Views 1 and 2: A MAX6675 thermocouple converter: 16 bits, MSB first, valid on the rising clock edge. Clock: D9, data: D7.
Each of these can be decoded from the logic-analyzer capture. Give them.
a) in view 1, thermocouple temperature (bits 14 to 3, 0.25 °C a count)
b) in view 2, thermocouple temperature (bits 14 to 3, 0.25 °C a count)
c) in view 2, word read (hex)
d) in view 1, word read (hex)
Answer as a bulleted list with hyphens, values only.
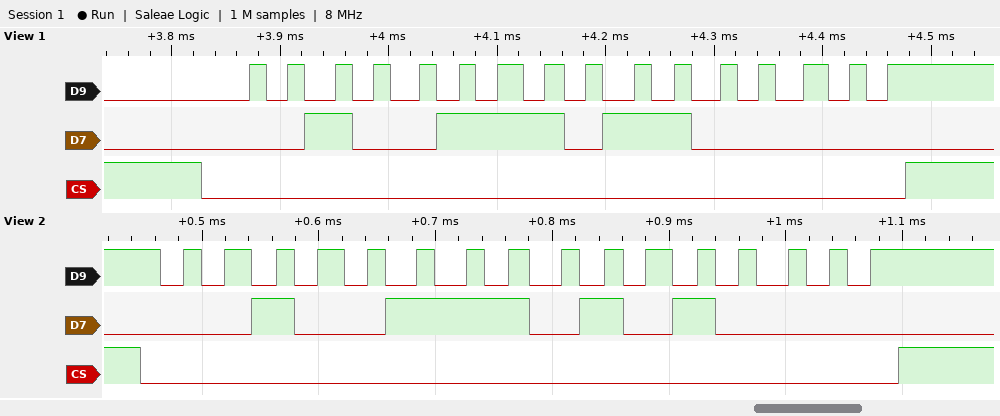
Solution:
- 315.00 °C
- 314.50 °C
- 0x2750
- 0x2760
